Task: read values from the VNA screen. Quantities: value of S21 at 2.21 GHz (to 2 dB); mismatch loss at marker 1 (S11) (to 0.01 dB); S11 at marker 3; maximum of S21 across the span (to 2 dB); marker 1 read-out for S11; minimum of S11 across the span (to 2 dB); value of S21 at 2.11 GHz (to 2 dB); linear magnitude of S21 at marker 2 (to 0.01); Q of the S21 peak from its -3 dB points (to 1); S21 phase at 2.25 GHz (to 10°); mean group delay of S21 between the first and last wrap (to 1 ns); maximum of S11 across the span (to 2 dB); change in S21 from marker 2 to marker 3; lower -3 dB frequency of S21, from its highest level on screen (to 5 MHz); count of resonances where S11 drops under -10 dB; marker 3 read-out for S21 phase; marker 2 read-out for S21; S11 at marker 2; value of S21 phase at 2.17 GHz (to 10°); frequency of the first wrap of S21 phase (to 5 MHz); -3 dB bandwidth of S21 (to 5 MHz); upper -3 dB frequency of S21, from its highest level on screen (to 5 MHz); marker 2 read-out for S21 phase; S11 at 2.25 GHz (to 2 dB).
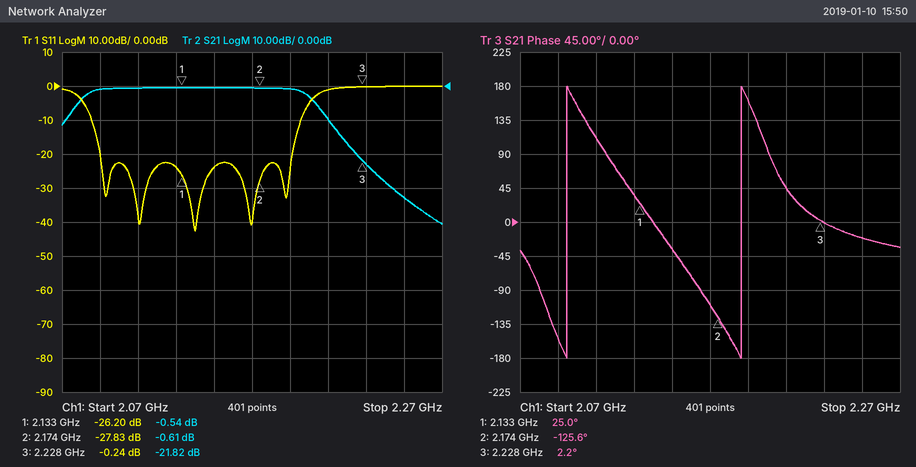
-10 dB
0.01 dB
-0.24 dB
0 dB
-26.20 dB
-42 dB
0 dB
0.93
18
-20°
11 ns
0 dB
-21.21 dB
2.080 GHz
5
2.2°
-0.61 dB
-27.83 dB
-110°
2.095 GHz
120 MHz
2.200 GHz
-125.6°
0 dB
